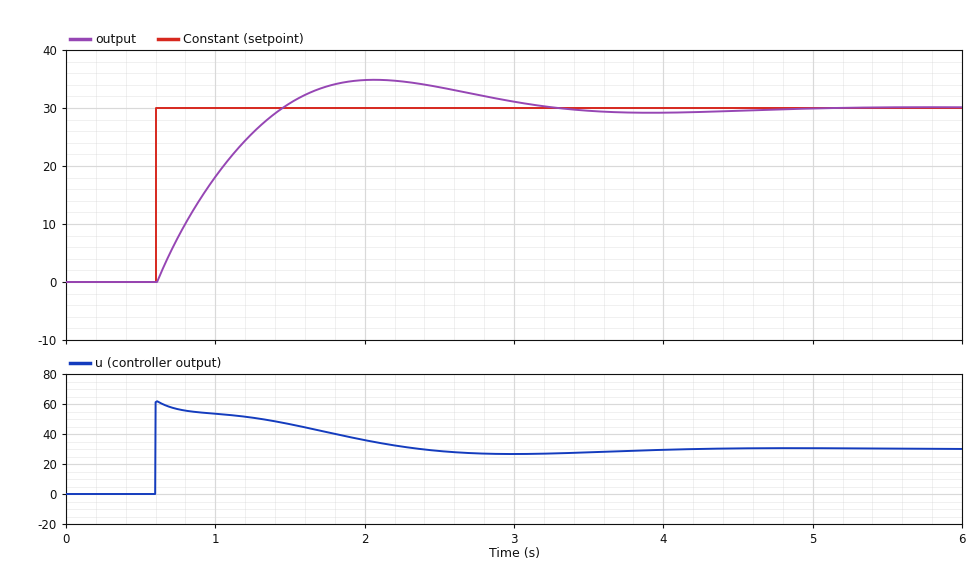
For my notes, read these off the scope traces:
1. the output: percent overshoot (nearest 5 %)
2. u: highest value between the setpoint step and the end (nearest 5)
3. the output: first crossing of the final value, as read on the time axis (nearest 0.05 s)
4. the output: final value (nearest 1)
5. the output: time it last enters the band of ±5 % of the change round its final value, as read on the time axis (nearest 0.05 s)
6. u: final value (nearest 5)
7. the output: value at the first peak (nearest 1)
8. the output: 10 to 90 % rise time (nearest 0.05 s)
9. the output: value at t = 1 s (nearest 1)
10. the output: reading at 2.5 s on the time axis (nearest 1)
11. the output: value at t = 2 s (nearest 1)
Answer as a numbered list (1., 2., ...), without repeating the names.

1. 15 %
2. 60
3. 1.45 s
4. 30
5. 2.90 s
6. 30
7. 35
8. 0.65 s
9. 18
10. 34
11. 35
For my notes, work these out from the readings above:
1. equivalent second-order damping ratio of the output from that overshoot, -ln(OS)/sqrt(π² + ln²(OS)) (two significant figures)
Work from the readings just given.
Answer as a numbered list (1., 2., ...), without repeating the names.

1. 0.52
